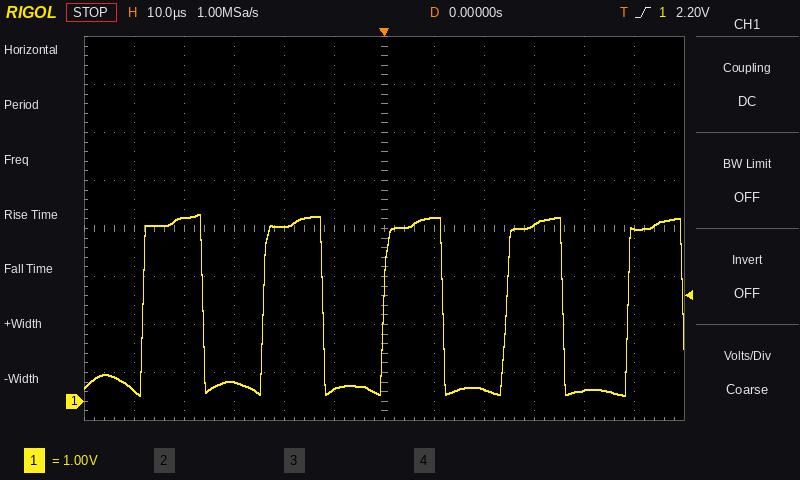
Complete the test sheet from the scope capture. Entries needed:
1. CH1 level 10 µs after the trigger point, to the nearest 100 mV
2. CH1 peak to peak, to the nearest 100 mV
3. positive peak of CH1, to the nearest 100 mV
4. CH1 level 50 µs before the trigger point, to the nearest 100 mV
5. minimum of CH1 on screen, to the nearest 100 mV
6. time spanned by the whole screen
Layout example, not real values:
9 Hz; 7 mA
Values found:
3.8 V; 3.8 V; 3.9 V; 200 mV; 100 mV; 120 µs
